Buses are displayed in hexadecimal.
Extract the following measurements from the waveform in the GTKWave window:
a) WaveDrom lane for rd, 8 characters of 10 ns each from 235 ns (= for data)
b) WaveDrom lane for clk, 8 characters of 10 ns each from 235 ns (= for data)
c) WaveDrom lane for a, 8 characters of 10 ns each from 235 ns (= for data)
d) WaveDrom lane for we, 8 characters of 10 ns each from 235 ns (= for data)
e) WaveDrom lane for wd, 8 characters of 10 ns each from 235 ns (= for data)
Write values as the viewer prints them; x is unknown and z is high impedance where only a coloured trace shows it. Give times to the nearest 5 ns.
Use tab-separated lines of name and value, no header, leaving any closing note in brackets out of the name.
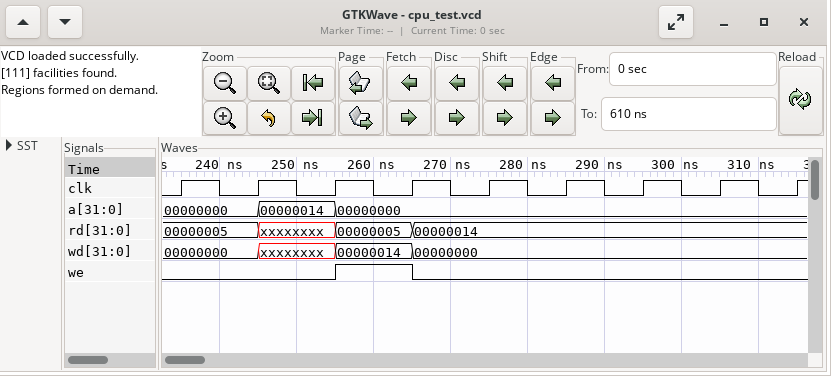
WaveDrom lane for rd, 8 characters of 10 ns each from 235 ns	{name: 'rd', wave: '=x==....', data: '00000005 00000005 00000014'}
WaveDrom lane for clk, 8 characters of 10 ns each from 235 ns	{name: 'clk', wave: 'p.......'}
WaveDrom lane for a, 8 characters of 10 ns each from 235 ns	{name: 'a', wave: '===.....', data: '00000000 00000014 00000000'}
WaveDrom lane for we, 8 characters of 10 ns each from 235 ns	{name: 'we', wave: '0.10....'}
WaveDrom lane for wd, 8 characters of 10 ns each from 235 ns	{name: 'wd', wave: '=x==....', data: '00000000 00000014 00000000'}
